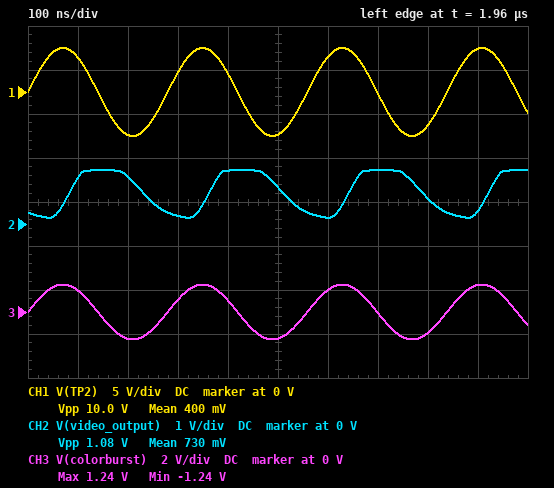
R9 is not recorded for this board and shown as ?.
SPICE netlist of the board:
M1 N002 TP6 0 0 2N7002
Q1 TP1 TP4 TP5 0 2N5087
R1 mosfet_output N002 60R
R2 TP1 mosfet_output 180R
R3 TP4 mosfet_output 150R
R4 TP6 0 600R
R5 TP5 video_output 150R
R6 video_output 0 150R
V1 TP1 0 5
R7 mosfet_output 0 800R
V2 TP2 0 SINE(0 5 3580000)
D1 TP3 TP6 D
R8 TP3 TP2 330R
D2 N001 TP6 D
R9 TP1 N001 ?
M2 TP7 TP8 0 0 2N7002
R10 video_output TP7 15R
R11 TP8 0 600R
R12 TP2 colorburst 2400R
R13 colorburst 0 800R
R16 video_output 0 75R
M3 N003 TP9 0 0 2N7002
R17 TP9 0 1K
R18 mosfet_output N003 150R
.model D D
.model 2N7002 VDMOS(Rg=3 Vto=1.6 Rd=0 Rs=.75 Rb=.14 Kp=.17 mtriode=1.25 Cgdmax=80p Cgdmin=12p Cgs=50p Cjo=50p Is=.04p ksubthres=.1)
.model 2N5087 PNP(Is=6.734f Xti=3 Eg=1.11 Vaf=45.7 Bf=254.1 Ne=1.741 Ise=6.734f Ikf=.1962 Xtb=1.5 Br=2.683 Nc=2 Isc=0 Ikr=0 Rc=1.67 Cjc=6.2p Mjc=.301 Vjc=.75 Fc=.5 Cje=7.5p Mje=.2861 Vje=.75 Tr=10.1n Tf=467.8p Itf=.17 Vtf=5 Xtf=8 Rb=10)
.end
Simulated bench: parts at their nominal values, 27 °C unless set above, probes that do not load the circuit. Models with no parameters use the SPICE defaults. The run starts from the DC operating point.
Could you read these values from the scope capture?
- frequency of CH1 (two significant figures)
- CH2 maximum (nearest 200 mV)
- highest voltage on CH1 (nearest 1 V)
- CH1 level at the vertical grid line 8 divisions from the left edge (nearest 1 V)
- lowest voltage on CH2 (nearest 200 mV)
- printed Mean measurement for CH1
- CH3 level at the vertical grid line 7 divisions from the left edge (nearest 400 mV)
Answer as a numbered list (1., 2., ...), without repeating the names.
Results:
1. 3.6 MHz
2. 1.2 V
3. 5 V
4. -4 V
5. 200 mV
6. 400 mV
7. 0 V
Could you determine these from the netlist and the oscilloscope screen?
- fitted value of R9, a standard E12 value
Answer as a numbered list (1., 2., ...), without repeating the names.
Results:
1. 1.5 kΩ
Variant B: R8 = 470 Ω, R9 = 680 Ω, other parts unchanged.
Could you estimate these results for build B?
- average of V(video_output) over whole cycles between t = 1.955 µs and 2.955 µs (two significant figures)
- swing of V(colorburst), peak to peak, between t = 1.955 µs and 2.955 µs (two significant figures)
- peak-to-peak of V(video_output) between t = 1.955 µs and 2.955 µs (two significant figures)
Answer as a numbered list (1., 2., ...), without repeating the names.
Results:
1. 1.2 V
2. 2.5 V
3. 2.3 mV
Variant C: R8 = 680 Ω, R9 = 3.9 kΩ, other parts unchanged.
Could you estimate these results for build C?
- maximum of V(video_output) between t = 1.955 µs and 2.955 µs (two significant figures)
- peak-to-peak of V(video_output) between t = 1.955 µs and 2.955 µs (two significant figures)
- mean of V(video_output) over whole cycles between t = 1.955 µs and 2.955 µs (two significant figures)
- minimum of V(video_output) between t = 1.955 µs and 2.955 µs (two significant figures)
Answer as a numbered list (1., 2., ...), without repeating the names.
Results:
1. 310 mV
2. 230 mV
3. 150 mV
4. 82 mV
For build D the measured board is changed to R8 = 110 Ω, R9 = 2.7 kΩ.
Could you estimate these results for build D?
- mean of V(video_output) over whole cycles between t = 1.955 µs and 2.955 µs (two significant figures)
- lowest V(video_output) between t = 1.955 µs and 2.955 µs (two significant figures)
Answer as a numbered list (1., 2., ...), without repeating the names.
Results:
1. 870 mV
2. 160 mV
